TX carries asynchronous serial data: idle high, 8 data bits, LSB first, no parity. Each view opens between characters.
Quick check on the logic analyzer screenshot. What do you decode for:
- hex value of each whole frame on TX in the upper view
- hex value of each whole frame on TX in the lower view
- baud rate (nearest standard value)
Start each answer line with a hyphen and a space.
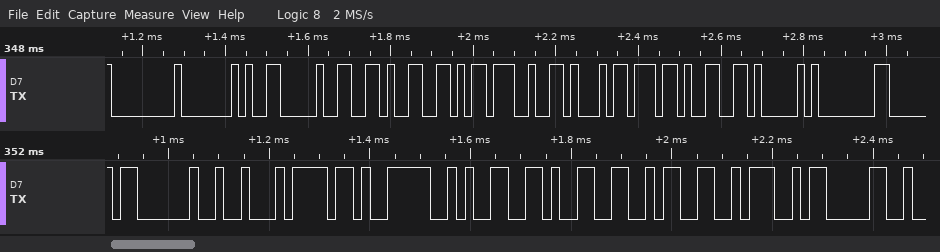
- 00, 40, 06, 66, 66, 3B, 16, BB, 99, 41, 80
- 03, 12, 6F, 3E, 99, 99, 9A, 3A, 83
- 57600 baud
